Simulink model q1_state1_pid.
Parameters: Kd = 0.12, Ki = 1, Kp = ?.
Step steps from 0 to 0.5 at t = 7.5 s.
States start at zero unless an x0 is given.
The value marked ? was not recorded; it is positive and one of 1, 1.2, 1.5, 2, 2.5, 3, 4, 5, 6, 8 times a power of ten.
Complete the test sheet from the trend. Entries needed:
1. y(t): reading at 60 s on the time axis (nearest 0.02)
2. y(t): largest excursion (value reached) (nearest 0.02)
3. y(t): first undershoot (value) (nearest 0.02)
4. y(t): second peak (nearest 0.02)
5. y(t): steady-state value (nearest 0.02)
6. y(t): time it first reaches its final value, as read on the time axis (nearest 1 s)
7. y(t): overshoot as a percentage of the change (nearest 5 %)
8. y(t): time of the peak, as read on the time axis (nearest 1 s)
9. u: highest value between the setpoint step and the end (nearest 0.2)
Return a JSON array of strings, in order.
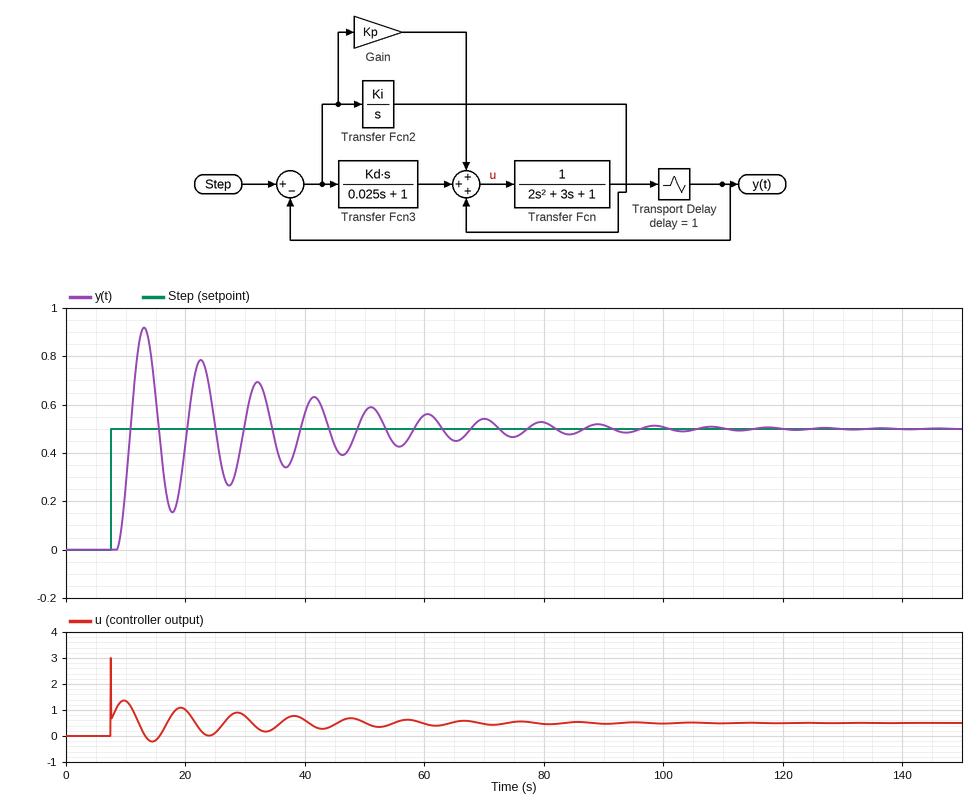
["0.56", "0.92", "0.16", "0.78", "0.50", "11 s", "85 %", "13 s", "3.0"]
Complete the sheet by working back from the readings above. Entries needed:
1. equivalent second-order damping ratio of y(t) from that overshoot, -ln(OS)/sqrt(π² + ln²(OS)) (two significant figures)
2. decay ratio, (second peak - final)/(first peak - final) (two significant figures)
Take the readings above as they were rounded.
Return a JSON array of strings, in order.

["0.052", "0.67"]
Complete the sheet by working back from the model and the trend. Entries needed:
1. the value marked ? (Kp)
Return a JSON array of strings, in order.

["1.2"]
